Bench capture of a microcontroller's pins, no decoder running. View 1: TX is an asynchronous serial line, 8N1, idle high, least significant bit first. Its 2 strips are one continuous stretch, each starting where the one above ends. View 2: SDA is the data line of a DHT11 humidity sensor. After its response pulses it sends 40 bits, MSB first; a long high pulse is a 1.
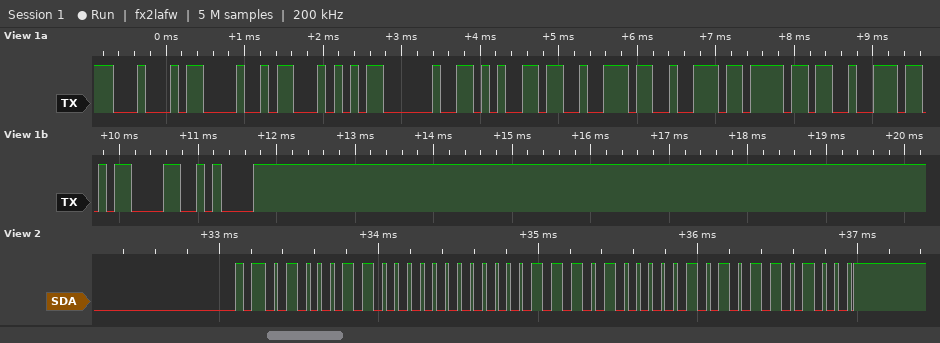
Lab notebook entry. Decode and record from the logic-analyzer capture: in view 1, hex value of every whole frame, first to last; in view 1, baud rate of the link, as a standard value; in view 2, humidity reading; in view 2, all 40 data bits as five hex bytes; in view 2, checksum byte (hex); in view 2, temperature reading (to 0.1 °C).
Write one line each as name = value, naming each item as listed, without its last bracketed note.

in view 1, hex value of every whole frame, first to last = 44 48 54 20 65 72 72 6F 72 0D 0A
in view 1, baud rate of the link, as a standard value = 9600 baud
in view 2, humidity reading = 70 %
in view 2, all 40 data bits as five hex bytes = 46 00 1D 05 68
in view 2, checksum byte = 0x68
in view 2, temperature reading = 29.5 °C
